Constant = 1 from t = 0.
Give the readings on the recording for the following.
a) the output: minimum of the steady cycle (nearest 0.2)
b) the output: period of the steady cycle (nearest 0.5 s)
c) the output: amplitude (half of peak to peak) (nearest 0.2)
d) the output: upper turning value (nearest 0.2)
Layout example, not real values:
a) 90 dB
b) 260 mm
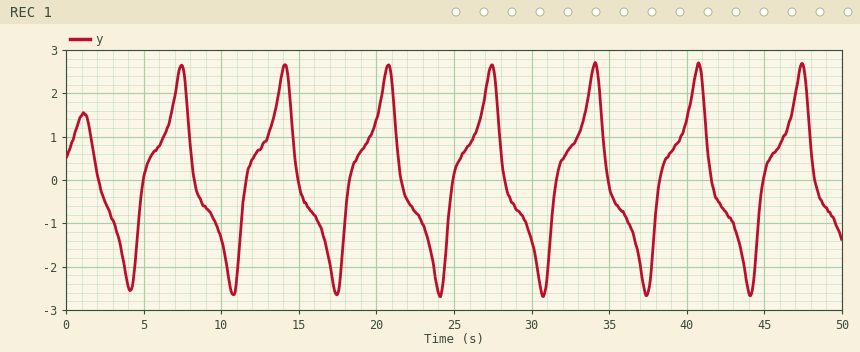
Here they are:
a) -2.6
b) 6.5 s
c) 2.6
d) 2.6
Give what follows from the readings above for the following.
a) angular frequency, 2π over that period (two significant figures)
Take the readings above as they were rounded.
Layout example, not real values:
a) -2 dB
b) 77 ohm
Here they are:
a) 0.97 rad/s
